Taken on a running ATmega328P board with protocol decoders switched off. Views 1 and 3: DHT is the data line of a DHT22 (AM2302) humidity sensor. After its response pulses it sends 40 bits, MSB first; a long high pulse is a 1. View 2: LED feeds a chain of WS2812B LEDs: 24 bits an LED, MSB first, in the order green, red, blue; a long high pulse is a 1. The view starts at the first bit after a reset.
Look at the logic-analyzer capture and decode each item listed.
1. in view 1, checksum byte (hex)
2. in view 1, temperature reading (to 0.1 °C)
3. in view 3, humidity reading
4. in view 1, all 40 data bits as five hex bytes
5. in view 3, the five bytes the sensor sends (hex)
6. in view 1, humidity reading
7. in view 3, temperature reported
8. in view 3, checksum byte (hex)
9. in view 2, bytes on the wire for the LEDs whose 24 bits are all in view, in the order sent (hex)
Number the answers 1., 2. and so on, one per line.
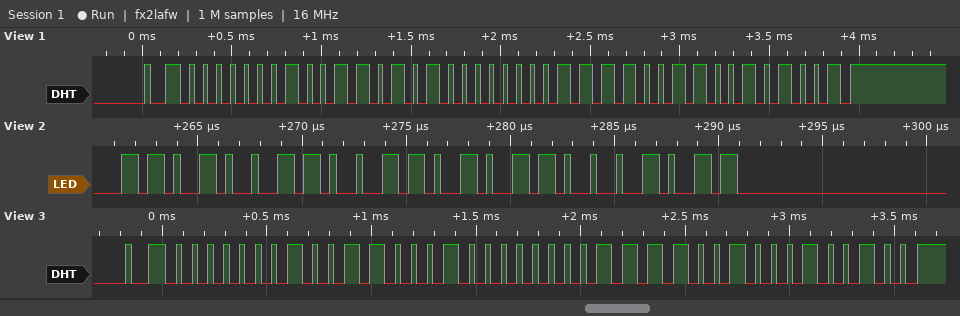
1. 0x29
2. 24.3 °C
3. 30.5 %
4. 01 35 00 F3 29
5. 01 31 00 F2 24
6. 30.9 %
7. 24.2 °C
8. 0x24
9. D3 35 8B
